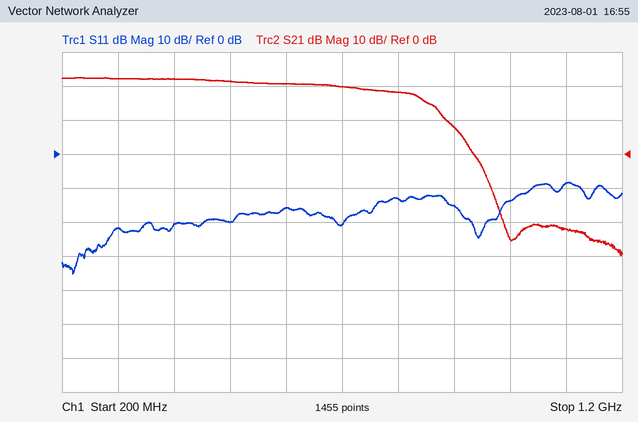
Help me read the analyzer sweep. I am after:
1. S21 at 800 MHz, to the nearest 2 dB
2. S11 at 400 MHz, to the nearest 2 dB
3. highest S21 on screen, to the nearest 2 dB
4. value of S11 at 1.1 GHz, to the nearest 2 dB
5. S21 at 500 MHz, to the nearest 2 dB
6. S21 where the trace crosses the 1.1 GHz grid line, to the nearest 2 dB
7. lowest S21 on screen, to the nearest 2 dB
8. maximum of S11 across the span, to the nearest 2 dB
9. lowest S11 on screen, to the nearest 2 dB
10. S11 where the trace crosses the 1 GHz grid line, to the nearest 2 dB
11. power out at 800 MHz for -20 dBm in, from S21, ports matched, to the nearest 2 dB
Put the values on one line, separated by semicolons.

18 dB; -20 dB; 22 dB; -8 dB; 22 dB; -22 dB; -30 dB; -8 dB; -36 dB; -14 dB; -2 dBm
